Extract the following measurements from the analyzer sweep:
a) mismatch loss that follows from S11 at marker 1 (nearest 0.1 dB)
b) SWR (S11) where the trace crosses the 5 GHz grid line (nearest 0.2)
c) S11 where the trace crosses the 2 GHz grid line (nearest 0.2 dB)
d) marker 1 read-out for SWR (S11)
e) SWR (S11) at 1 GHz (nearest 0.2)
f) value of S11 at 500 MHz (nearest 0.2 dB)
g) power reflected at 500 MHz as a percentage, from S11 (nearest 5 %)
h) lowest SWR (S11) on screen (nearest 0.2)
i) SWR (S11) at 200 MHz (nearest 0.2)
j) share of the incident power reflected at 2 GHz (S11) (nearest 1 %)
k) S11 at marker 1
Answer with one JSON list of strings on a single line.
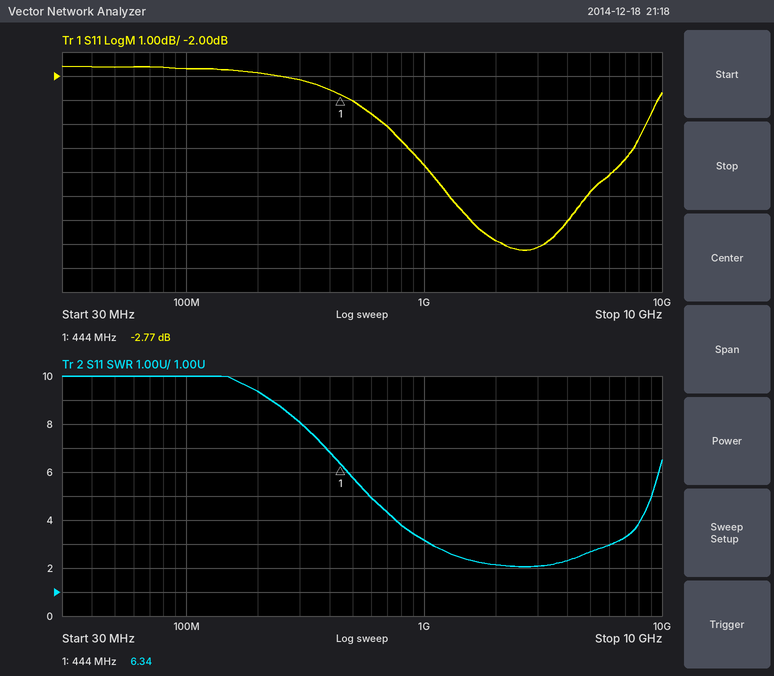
["3.3 dB", "2.6", "-8.8 dB", "6.34", "3.2", "-3.0 dB", "50 %", "2.0", "9.4", "13 %", "-2.77 dB"]
